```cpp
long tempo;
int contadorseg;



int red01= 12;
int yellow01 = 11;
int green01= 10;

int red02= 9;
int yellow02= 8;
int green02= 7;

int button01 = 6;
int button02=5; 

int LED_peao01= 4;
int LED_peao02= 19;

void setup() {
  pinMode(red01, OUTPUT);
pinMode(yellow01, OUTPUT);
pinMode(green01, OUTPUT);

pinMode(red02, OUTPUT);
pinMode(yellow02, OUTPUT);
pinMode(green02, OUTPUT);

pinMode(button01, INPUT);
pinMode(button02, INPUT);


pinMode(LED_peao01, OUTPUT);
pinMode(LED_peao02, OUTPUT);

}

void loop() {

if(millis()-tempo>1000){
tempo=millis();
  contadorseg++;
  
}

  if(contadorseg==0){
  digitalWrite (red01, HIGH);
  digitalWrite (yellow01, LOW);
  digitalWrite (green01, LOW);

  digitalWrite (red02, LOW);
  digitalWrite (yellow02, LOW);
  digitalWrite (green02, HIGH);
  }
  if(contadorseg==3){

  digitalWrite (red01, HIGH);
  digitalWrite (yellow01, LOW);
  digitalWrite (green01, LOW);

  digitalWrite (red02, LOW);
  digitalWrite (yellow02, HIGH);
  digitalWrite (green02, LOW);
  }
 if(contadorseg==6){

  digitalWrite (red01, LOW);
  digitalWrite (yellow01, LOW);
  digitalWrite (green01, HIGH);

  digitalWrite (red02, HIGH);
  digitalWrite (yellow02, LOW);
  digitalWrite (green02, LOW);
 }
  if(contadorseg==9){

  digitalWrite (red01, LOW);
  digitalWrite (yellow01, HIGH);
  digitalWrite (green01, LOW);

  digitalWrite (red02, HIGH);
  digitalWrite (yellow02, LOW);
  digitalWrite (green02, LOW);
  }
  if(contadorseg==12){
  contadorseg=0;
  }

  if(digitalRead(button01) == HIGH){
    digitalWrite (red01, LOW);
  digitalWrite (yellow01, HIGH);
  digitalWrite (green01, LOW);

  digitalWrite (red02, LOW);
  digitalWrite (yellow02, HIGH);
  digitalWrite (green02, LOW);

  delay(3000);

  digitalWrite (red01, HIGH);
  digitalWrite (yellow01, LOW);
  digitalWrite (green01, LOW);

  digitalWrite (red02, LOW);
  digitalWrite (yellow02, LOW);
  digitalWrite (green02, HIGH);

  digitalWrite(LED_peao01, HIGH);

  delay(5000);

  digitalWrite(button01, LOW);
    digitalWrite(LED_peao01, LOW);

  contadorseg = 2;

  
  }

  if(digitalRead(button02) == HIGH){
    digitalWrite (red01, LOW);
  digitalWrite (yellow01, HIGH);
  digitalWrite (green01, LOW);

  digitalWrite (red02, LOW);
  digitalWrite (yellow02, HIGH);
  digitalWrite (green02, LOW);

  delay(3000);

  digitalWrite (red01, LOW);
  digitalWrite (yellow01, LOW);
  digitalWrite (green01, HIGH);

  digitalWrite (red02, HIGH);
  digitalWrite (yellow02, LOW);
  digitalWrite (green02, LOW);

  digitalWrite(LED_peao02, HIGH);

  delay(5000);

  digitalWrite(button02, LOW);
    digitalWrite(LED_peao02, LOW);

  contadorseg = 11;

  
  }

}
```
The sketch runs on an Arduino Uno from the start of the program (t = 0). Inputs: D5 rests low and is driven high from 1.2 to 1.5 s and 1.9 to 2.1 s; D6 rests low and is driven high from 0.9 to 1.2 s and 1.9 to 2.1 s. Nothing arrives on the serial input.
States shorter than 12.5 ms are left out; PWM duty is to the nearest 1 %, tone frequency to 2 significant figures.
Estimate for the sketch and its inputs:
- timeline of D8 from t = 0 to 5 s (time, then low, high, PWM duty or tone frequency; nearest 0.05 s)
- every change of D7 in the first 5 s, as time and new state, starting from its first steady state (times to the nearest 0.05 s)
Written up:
0 s low; 0.9 s high; 3.9 s low
0 s high; 0.9 s low; 3.9 s high
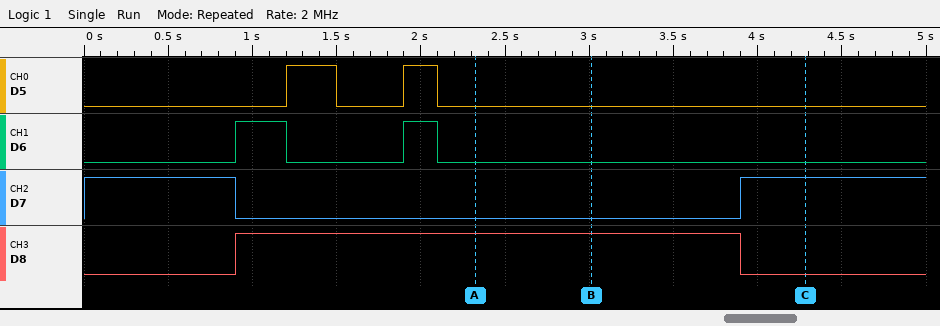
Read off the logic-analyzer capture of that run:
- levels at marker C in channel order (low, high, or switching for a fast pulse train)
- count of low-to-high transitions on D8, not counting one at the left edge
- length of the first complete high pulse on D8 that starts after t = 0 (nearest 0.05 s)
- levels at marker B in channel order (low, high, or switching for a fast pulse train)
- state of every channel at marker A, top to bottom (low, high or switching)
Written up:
D5 low, D6 low, D7 high, D8 low
1
3.00 s
D5 low, D6 low, D7 low, D8 high
D5 low, D6 low, D7 low, D8 high
